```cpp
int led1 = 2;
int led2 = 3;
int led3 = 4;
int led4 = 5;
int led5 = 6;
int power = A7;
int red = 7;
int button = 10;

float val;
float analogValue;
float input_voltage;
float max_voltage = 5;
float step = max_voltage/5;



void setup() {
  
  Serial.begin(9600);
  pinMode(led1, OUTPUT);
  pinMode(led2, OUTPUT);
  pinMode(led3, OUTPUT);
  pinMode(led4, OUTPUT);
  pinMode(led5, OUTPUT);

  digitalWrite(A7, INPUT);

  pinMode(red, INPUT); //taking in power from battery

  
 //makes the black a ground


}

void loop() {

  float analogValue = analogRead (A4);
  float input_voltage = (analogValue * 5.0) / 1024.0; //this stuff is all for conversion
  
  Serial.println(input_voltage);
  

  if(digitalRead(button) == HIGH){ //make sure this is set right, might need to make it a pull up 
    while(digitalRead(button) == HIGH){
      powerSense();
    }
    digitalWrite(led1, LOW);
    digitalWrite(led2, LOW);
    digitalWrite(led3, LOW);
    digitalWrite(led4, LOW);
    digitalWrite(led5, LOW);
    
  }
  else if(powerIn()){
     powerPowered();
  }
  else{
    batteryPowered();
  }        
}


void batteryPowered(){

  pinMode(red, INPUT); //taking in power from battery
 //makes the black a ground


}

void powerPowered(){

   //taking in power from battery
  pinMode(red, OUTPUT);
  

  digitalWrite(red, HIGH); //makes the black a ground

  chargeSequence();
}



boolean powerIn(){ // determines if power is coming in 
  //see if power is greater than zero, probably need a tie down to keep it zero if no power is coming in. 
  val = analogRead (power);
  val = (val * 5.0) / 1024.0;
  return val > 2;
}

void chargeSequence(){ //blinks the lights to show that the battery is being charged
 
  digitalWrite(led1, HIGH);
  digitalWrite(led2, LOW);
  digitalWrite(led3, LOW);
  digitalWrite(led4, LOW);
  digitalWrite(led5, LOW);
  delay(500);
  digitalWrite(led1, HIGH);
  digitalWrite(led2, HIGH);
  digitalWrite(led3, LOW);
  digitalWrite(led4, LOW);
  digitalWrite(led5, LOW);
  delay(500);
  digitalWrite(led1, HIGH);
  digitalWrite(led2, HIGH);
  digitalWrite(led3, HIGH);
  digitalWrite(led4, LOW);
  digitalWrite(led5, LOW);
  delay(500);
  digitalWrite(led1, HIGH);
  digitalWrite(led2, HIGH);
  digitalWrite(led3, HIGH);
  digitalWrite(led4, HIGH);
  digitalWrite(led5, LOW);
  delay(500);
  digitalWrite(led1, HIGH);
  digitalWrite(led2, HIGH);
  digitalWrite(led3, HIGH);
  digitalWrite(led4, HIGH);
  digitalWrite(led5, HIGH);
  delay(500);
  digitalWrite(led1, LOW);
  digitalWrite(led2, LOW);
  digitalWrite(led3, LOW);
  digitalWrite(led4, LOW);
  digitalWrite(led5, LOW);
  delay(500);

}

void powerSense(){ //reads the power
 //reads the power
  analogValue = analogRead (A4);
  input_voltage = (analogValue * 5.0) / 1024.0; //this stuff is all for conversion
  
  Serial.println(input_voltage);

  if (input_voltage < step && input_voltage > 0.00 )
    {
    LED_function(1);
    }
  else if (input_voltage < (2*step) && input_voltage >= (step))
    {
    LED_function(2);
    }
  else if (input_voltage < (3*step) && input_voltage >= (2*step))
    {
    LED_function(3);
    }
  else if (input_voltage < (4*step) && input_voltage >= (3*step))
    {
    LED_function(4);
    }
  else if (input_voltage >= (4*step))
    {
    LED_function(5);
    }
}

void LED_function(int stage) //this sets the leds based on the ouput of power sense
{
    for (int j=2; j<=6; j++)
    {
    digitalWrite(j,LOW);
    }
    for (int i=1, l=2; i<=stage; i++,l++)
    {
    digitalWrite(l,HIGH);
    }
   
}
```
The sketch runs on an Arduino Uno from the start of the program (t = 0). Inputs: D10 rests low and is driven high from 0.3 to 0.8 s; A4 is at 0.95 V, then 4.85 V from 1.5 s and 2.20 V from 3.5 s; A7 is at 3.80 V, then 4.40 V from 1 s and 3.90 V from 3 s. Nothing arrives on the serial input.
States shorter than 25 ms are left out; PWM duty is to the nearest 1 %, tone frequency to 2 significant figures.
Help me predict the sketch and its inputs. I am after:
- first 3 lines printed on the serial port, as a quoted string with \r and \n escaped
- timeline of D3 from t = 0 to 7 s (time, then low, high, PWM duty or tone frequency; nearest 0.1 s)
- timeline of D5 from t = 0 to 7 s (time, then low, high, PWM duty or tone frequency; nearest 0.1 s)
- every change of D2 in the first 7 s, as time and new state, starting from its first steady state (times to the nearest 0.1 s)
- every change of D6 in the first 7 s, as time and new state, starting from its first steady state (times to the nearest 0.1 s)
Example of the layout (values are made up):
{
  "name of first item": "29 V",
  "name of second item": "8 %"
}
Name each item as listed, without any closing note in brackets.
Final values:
{
  "first 3 lines printed on the serial port, as a quoted string with \\r and \\n escaped": "\"0.95\\r\\n4.85\\r\\n2.20\\r\\n\"",
  "timeline of D3 from t = 0 to 7 s": "0 s low; 0.5 s high; 2.5 s low; 3.5 s high; 5.5 s low; 6.5 s high",
  "timeline of D5 from t = 0 to 7 s": "0 s low; 1.5 s high; 2.5 s low; 4.5 s high; 5.5 s low",
  "every change of D2 in the first 7 s, as time and new state, starting from its first steady state": "0 s high; 2.5 s low; 3 s high; 5.5 s low; 6 s high",
  "every change of D6 in the first 7 s, as time and new state, starting from its first steady state": "0 s low; 2 s high; 2.5 s low; 5 s high; 5.5 s low"
}
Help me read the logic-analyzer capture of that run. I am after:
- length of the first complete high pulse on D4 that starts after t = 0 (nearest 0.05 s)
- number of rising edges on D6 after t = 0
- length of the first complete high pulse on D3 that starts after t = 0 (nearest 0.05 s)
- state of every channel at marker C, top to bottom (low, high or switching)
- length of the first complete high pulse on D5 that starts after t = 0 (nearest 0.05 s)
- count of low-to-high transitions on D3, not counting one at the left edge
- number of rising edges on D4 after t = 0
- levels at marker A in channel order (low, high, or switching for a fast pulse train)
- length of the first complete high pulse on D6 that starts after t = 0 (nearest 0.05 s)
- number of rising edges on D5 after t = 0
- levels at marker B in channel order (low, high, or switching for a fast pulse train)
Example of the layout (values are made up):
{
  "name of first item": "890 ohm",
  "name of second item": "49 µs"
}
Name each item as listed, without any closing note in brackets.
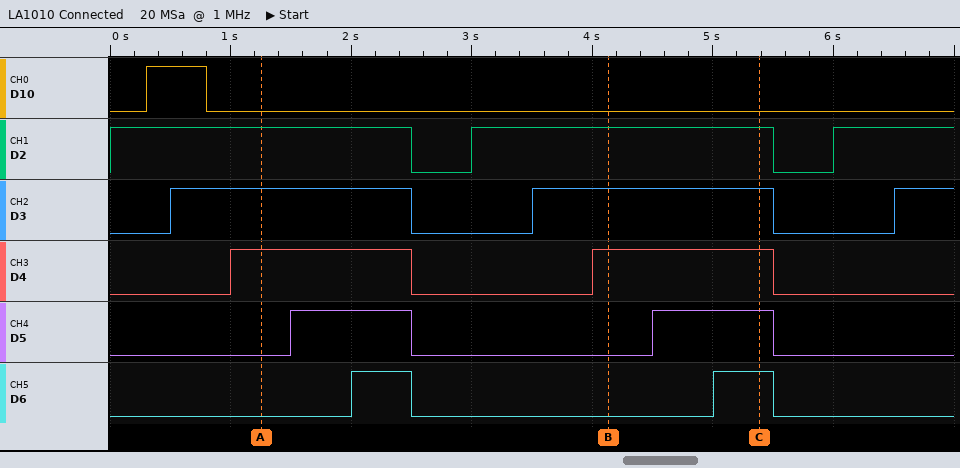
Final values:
{
  "length of the first complete high pulse on D4 that starts after t = 0": "1.50 s",
  "number of rising edges on D6 after t = 0": "2",
  "length of the first complete high pulse on D3 that starts after t = 0": "2.00 s",
  "state of every channel at marker C, top to bottom": "D10 low, D2 high, D3 high, D4 high, D5 high, D6 high",
  "length of the first complete high pulse on D5 that starts after t = 0": "1.00 s",
  "count of low-to-high transitions on D3, not counting one at the left edge": "3",
  "number of rising edges on D4 after t = 0": "2",
  "levels at marker A in channel order": "D10 low, D2 high, D3 high, D4 high, D5 low, D6 low",
  "length of the first complete high pulse on D6 that starts after t = 0": "0.50 s",
  "number of rising edges on D5 after t = 0": "2",
  "levels at marker B in channel order": "D10 low, D2 high, D3 high, D4 high, D5 low, D6 low"
}
